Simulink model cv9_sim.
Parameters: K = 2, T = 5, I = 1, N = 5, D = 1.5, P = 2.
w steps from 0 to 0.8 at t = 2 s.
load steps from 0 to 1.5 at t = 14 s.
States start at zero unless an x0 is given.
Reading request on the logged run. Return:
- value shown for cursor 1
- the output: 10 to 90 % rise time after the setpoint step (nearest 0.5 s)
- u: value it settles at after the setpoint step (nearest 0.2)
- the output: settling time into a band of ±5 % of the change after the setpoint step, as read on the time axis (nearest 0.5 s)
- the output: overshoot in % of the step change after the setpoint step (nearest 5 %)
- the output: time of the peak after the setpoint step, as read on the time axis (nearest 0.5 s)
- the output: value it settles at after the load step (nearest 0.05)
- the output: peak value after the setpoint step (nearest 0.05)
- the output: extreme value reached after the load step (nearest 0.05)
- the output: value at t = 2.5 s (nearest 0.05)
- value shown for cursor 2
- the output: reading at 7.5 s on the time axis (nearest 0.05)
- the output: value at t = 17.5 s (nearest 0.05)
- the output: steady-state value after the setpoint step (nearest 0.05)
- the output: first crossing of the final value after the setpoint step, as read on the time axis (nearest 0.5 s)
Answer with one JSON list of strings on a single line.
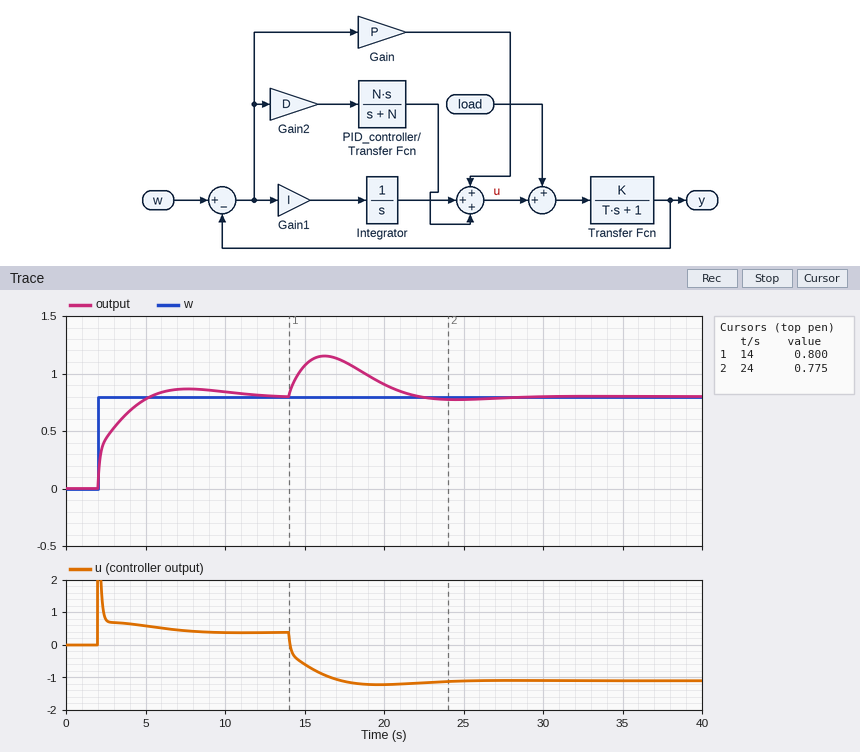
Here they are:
["0.800", "2.5 s", "0.4", "10.0 s", "10 %", "7.5 s", "0.80", "0.85", "1.15", "0.45", "0.775", "0.85", "1.10", "0.80", "5.5 s"]
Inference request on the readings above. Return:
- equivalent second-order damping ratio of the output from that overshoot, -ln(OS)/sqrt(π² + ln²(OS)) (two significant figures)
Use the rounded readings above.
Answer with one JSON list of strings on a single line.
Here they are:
["0.59"]
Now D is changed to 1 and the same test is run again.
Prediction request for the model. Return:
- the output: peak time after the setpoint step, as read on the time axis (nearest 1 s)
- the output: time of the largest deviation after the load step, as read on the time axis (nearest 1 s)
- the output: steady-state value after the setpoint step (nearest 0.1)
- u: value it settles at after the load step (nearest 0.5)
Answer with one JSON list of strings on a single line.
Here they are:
["7 s", "16 s", "0.8", "-1.0"]
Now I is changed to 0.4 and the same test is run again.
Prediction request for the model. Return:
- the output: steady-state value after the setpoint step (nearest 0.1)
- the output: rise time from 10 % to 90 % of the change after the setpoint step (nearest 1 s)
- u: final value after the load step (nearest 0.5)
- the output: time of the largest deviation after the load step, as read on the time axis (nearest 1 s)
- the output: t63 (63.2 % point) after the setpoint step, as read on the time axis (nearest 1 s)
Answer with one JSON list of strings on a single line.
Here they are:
["0.8", "4 s", "-1.0", "17 s", "3 s"]
